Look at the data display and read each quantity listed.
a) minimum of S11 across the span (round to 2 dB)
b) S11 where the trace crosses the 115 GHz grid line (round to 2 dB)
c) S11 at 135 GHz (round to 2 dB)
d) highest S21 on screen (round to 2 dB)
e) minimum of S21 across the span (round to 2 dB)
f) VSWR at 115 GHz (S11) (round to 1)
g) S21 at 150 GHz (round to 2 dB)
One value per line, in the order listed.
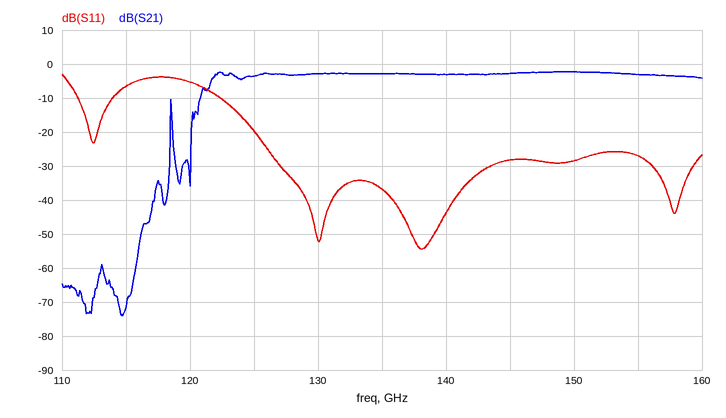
-54 dB
-6 dB
-36 dB
-2 dB
-74 dB
3
-2 dB
